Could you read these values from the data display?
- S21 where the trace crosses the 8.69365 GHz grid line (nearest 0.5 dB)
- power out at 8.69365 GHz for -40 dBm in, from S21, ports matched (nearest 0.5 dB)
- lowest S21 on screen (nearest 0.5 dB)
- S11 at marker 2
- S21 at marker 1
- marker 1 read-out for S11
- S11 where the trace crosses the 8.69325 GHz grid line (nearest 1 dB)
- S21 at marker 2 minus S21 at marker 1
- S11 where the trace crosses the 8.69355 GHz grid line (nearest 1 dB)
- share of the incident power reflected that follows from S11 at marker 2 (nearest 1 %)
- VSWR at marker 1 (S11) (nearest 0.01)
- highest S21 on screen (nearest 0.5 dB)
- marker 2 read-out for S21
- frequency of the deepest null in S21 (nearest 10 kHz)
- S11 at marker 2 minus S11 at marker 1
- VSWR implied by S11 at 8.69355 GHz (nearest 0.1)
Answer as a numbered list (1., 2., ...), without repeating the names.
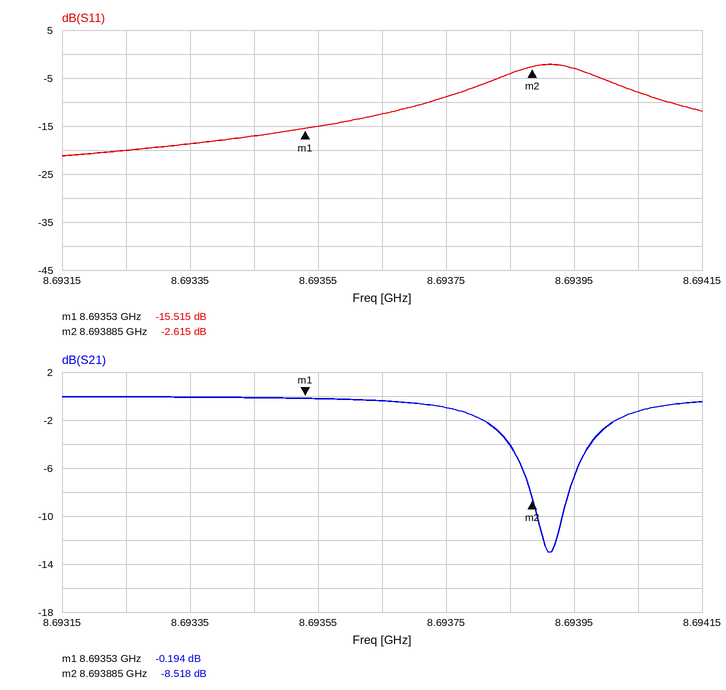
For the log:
1. -0.5 dB
2. -40.5 dBm
3. -13.0 dB
4. -2.615 dB
5. -0.194 dB
6. -15.515 dB
7. -20 dB
8. -8.324 dB
9. -15 dB
10. 55 %
11. 1.40
12. 0.0 dB
13. -8.518 dB
14. 8.69391 GHz
15. 12.900 dB
16. 1.4
